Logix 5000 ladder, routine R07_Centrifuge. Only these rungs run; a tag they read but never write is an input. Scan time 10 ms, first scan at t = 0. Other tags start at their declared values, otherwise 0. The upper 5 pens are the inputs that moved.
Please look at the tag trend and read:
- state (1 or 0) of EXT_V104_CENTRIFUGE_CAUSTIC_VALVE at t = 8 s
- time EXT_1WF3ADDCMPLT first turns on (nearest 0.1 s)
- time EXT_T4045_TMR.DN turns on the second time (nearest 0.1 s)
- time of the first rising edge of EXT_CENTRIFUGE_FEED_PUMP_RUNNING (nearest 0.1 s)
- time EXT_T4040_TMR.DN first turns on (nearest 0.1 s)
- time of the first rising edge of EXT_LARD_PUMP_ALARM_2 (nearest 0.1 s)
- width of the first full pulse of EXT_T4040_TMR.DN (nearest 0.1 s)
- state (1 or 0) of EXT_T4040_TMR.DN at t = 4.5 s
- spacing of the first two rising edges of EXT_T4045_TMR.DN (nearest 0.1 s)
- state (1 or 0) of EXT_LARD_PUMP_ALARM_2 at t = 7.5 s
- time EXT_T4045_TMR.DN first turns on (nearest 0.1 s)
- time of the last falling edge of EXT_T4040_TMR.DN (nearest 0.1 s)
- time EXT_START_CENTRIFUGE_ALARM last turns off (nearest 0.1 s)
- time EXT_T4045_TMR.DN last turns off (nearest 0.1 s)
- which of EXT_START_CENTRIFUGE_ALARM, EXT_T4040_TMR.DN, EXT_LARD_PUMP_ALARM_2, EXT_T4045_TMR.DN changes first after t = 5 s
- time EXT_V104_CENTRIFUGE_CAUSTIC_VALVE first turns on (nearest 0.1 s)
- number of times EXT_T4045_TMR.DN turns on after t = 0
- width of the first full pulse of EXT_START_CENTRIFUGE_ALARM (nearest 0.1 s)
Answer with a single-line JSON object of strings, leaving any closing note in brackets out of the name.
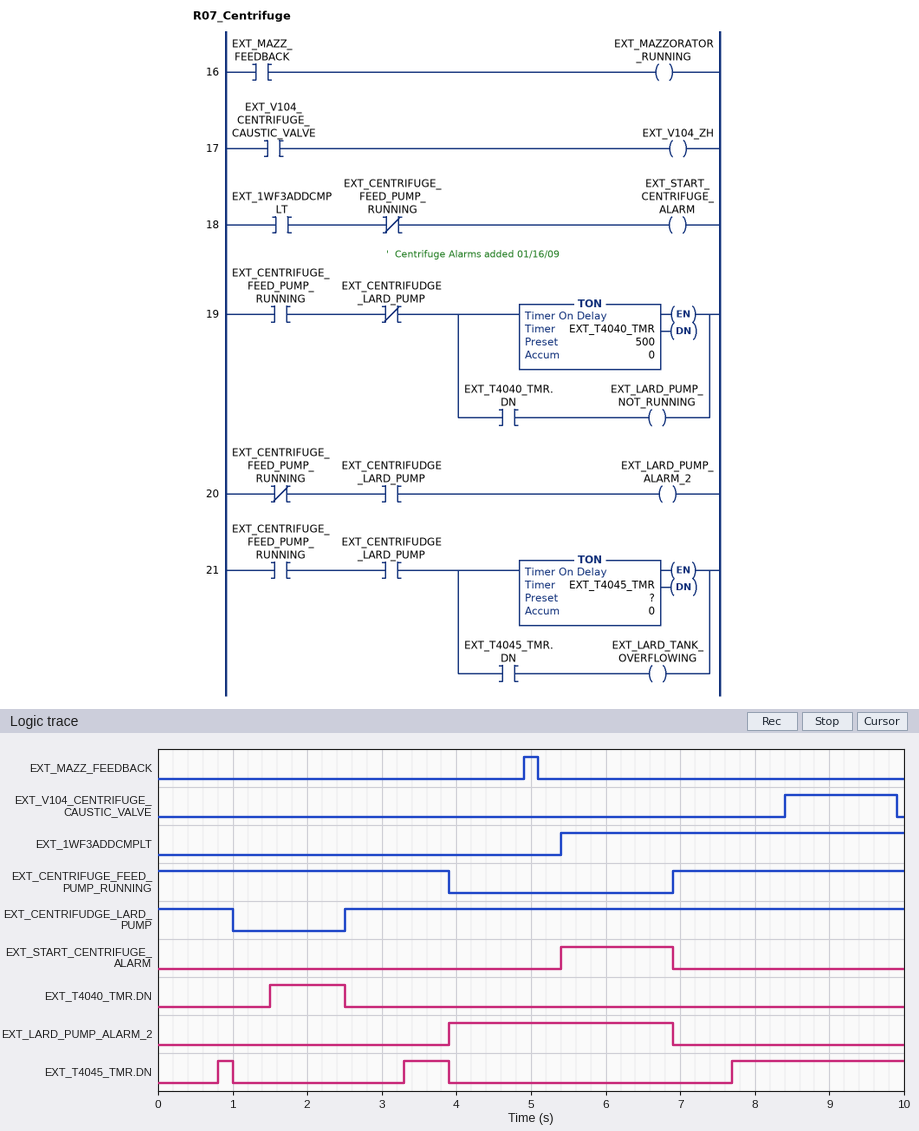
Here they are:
{"state (1 or 0) of EXT_V104_CENTRIFUGE_CAUSTIC_VALVE at t = 8 s": "0", "time EXT_1WF3ADDCMPLT first turns on": "5.4 s", "time EXT_T4045_TMR.DN turns on the second time": "3.3 s", "time of the first rising edge of EXT_CENTRIFUGE_FEED_PUMP_RUNNING": "6.9 s", "time EXT_T4040_TMR.DN first turns on": "1.5 s", "time of the first rising edge of EXT_LARD_PUMP_ALARM_2": "3.9 s", "width of the first full pulse of EXT_T4040_TMR.DN": "1.0 s", "state (1 or 0) of EXT_T4040_TMR.DN at t = 4.5 s": "0", "spacing of the first two rising edges of EXT_T4045_TMR.DN": "2.5 s", "state (1 or 0) of EXT_LARD_PUMP_ALARM_2 at t = 7.5 s": "0", "time EXT_T4045_TMR.DN first turns on": "0.8 s", "time of the last falling edge of EXT_T4040_TMR.DN": "2.5 s", "time EXT_START_CENTRIFUGE_ALARM last turns off": "6.9 s", "time EXT_T4045_TMR.DN last turns off": "3.9 s", "which of EXT_START_CENTRIFUGE_ALARM, EXT_T4040_TMR.DN, EXT_LARD_PUMP_ALARM_2, EXT_T4045_TMR.DN changes first after t = 5 s": "EXT_START_CENTRIFUGE_ALARM", "time EXT_V104_CENTRIFUGE_CAUSTIC_VALVE first turns on": "8.4 s", "number of times EXT_T4045_TMR.DN turns on after t = 0": "3", "width of the first full pulse of EXT_START_CENTRIFUGE_ALARM": "1.5 s"}
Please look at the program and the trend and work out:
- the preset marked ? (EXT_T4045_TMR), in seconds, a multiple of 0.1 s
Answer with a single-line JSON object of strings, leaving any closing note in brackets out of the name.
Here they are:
{"the preset marked ? (EXT_T4045_TMR), in seconds, a multiple of 0.1 s": "0.8 s"}
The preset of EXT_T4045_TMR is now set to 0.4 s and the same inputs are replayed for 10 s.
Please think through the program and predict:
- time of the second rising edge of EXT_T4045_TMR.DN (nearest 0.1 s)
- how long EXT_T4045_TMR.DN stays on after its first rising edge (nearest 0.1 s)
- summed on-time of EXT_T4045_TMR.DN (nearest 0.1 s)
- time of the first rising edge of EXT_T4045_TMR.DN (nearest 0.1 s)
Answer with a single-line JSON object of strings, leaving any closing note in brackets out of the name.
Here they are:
{"time of the second rising edge of EXT_T4045_TMR.DN": "2.9 s", "how long EXT_T4045_TMR.DN stays on after its first rising edge": "0.6 s", "summed on-time of EXT_T4045_TMR.DN": "4.3 s", "time of the first rising edge of EXT_T4045_TMR.DN": "0.4 s"}
